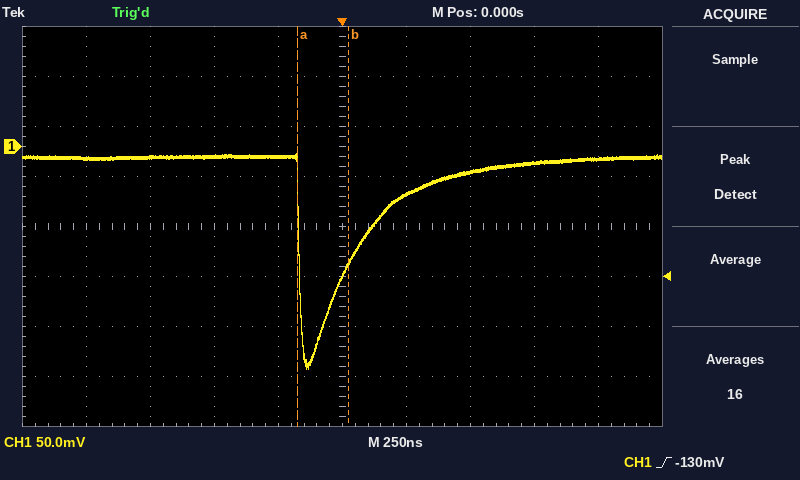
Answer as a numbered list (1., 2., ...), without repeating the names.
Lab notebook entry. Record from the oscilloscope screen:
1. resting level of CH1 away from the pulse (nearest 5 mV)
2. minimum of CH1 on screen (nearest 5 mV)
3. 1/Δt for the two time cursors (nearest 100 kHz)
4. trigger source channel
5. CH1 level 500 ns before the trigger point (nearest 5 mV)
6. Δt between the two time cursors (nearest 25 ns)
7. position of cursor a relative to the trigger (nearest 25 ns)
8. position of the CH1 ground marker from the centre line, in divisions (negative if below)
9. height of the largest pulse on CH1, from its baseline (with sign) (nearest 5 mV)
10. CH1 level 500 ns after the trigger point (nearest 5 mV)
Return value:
1. -10 mV
2. -220 mV
3. 5.0 MHz
4. CH1
5. -10 mV
6. 200 ns
7. -175 ns
8. +1.6 div
9. -210 mV
10. -25 mV
